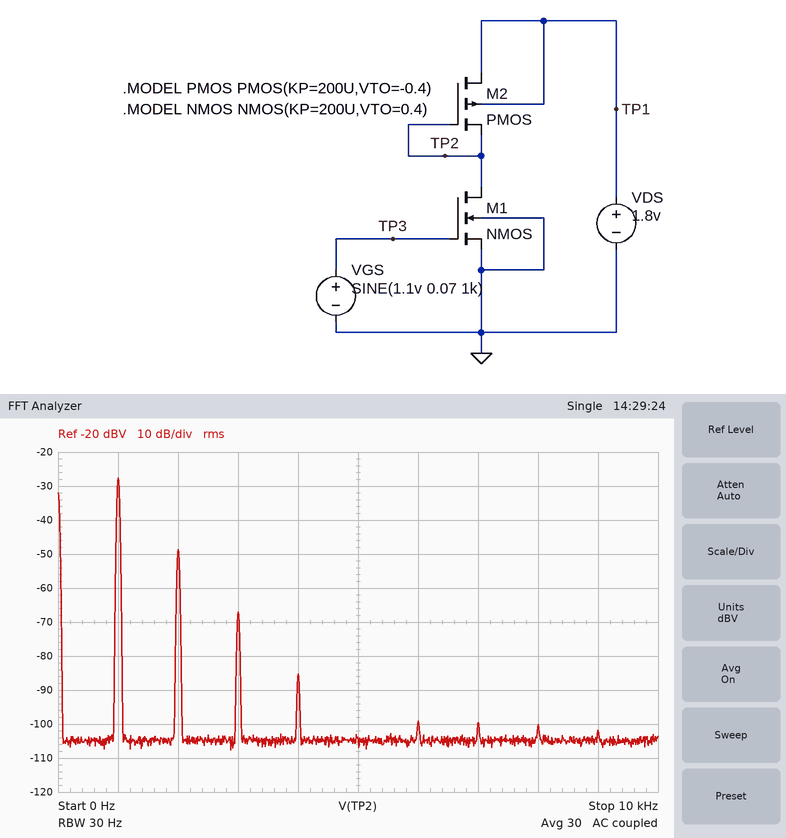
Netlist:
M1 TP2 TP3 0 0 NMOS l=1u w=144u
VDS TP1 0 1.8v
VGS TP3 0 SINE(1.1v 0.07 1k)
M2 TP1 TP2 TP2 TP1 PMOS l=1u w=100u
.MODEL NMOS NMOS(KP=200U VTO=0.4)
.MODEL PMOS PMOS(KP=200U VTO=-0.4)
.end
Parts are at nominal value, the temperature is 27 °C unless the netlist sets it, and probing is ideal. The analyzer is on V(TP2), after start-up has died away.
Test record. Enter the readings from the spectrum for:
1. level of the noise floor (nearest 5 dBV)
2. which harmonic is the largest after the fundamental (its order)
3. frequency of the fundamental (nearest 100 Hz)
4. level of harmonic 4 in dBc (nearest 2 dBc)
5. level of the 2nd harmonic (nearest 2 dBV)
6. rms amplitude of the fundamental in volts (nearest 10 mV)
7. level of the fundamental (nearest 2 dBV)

-105 dBV
2
1.0 kHz
-58 dBc
-48 dBV
40 mV
-28 dBV
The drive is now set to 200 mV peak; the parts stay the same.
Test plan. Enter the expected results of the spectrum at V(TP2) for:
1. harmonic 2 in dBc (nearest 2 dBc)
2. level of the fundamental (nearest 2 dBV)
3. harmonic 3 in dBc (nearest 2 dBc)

-16 dBc
-18 dBV
-50 dBc
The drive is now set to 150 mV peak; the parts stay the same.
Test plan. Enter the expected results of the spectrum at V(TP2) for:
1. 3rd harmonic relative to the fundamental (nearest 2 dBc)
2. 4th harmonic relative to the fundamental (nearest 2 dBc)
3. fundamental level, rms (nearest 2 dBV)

-50 dBc
-38 dBc
-20 dBV
